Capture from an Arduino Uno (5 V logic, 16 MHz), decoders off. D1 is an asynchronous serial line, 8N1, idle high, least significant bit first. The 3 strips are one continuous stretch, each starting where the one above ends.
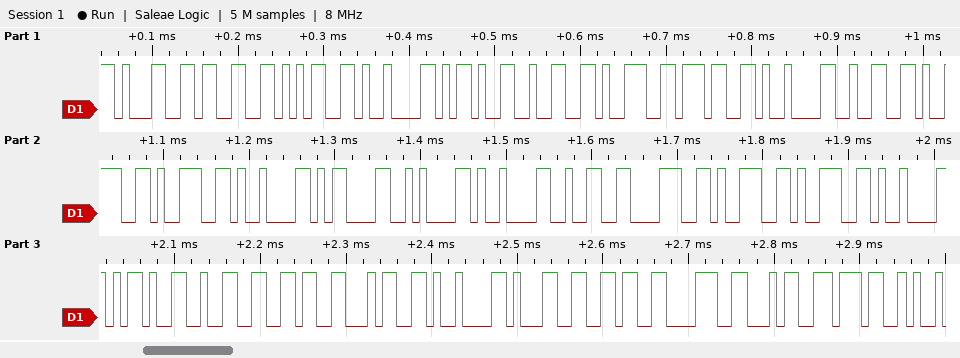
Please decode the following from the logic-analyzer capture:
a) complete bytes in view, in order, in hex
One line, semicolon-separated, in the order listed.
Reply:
31 33 35 09 2D 32 39 37 09 32 39 39 09 0D 0A 09 32 38 39 39 09 2D 32 36 34 09 31 36 38 34 37
